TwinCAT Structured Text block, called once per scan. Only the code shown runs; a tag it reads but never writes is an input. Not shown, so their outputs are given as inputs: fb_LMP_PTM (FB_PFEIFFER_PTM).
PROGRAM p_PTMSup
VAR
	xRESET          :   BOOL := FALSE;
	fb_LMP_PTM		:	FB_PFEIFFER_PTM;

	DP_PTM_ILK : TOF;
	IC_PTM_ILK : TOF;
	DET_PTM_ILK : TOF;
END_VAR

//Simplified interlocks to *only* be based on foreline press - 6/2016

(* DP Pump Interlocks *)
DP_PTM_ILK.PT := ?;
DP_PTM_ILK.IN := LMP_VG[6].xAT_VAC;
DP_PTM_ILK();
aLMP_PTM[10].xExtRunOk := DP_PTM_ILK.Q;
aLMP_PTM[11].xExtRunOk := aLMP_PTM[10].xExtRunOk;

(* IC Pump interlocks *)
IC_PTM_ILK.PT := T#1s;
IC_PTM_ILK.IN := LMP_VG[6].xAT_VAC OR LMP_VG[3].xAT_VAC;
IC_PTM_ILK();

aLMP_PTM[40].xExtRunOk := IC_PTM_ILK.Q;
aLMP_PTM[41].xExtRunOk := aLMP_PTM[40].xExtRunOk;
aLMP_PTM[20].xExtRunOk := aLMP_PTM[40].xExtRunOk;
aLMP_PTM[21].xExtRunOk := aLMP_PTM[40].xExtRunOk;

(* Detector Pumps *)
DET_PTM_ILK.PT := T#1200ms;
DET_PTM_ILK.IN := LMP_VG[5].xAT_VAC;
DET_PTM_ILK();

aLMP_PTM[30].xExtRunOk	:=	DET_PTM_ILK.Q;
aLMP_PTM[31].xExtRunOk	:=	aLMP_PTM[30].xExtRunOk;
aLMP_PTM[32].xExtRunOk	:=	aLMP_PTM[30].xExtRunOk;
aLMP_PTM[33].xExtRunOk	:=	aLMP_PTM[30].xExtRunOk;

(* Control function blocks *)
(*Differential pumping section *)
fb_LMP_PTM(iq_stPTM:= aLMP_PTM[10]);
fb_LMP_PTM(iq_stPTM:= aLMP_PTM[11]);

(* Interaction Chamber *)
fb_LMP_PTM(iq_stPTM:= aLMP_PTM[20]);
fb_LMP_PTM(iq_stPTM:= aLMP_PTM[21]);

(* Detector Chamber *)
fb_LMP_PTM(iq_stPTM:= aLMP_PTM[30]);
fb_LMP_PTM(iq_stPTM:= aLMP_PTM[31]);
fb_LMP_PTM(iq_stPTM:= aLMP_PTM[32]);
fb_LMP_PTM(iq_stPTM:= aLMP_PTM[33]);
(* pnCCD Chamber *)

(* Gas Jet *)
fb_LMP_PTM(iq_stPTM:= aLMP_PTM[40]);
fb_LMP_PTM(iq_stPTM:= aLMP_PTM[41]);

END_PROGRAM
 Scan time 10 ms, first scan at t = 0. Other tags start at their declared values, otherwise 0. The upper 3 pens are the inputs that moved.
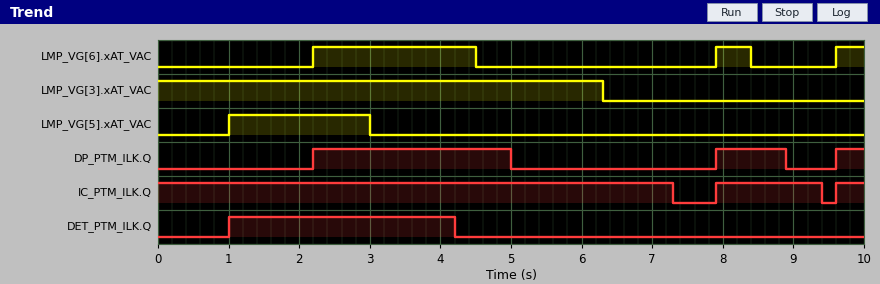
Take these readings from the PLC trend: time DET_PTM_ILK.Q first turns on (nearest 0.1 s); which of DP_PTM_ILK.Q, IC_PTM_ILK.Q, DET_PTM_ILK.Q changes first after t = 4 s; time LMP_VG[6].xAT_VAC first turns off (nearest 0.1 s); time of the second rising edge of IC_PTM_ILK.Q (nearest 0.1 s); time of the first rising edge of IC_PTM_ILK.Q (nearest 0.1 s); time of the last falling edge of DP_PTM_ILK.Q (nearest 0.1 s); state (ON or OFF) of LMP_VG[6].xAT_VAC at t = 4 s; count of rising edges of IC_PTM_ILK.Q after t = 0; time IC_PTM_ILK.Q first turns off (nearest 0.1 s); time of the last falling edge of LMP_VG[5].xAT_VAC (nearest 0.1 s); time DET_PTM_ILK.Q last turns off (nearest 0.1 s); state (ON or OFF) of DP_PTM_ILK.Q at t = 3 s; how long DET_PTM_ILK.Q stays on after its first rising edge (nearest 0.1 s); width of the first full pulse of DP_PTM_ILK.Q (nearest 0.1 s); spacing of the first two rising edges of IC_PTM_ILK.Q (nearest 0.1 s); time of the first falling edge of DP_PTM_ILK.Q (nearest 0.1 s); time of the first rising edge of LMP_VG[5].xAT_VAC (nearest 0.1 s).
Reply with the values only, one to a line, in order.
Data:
1.0 s
DET_PTM_ILK.Q
4.5 s
9.6 s
7.9 s
8.9 s
ON
2
7.3 s
3.0 s
4.2 s
ON
3.2 s
2.8 s
1.7 s
5.0 s
1.0 s
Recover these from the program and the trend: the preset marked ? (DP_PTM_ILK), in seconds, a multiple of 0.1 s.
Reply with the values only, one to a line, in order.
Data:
0.5 s
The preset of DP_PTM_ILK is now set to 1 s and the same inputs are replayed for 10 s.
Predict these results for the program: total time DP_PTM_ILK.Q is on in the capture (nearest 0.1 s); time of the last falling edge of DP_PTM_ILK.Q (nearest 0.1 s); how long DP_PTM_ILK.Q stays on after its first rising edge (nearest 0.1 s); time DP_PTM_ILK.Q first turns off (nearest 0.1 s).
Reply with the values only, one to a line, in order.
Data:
5.2 s
9.4 s
3.3 s
5.5 s
